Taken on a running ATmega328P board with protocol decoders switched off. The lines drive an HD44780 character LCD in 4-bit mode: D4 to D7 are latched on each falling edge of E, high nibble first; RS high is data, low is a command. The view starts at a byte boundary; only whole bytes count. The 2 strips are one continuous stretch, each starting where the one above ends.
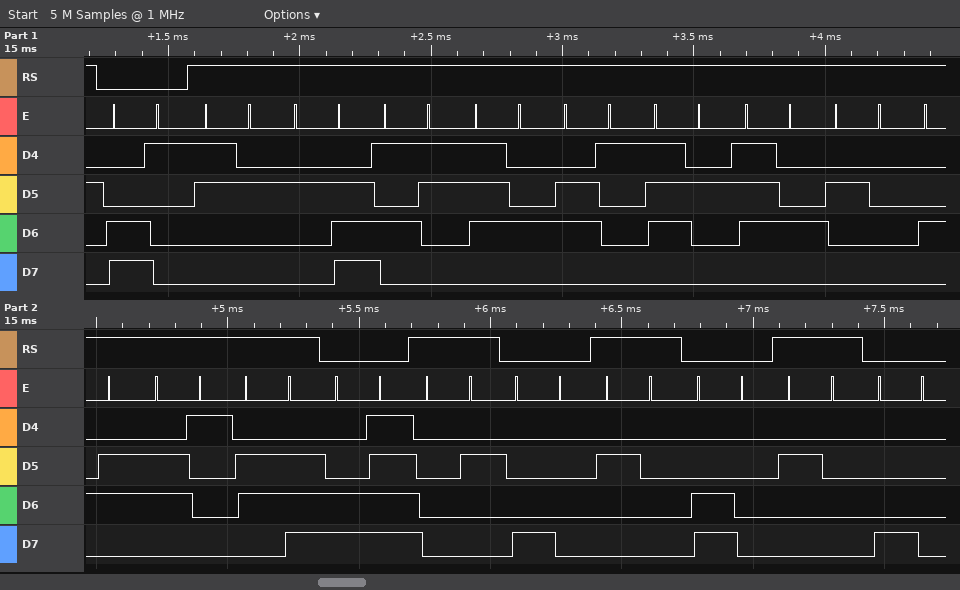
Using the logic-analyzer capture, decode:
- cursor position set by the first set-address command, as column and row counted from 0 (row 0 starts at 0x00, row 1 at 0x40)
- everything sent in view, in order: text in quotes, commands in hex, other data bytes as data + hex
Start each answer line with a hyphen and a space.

- column 1, row 1
- 0xC1 "2.Start Fan" 0xCF data 02 0x80 " " 0xC0 " " 0x80
